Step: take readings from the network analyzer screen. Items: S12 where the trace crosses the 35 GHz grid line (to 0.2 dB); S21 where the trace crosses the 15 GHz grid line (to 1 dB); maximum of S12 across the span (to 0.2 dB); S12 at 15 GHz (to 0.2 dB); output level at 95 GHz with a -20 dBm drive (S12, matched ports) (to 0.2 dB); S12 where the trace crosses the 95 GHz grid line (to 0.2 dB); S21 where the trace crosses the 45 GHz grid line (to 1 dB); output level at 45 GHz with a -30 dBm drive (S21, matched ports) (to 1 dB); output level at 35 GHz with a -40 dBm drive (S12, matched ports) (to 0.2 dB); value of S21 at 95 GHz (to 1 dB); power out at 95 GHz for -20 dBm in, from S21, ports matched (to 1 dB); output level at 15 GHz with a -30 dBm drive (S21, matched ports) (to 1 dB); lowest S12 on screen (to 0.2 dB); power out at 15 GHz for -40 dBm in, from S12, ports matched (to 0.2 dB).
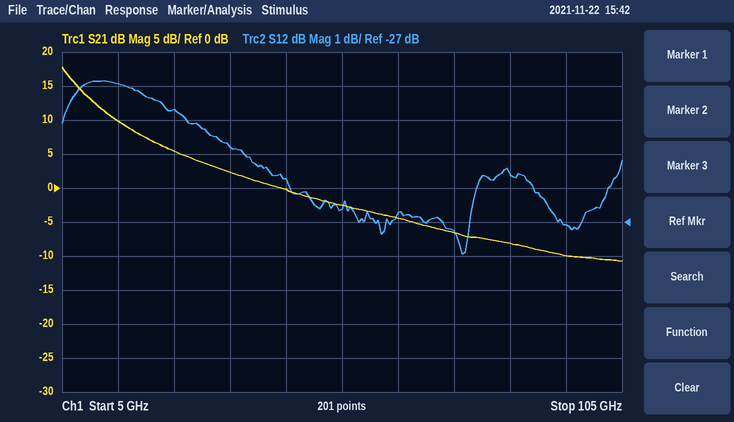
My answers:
-24.8 dB
10 dB
-22.8 dB
-23.0 dB
-47.0 dBm
-27.0 dB
0 dB
-30 dBm
-64.8 dBm
-10 dB
-30 dBm
-20 dBm
-28.0 dB
-63.0 dBm
